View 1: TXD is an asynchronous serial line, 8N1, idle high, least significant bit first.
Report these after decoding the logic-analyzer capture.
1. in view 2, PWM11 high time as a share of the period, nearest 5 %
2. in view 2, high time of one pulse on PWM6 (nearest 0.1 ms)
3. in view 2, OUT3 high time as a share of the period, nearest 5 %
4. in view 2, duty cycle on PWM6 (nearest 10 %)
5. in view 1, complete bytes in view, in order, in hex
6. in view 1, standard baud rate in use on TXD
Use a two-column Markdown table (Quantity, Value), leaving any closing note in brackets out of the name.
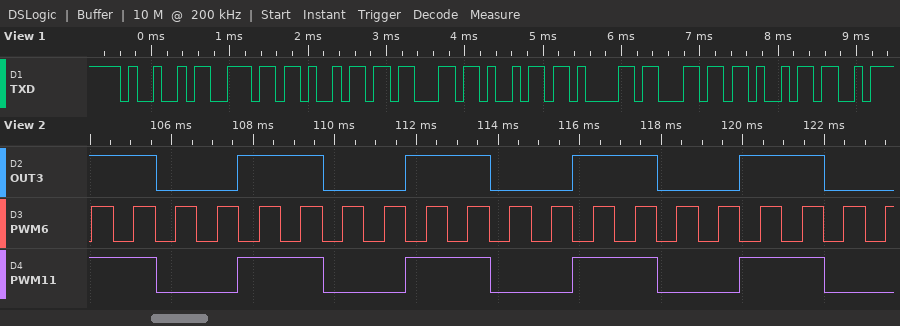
| Quantity | Value |
|---|---|
| in view 2, PWM11 high time as a share of the period, nearest 5 % | 50 % |
| in view 2, high time of one pulse on PWM6 | 0.5 ms |
| in view 2, OUT3 high time as a share of the period, nearest 5 % | 50 % |
| in view 2, duty cycle on PWM6 | 50 % |
| in view 1, complete bytes in view, in order, in hex | 49 6E 69 63 69 61 6C 69 |
| in view 1, standard baud rate in use on TXD | 9600 baud |
